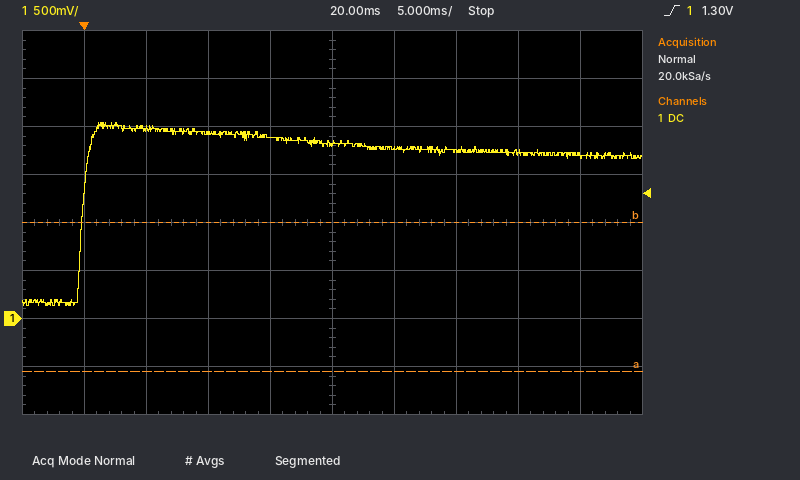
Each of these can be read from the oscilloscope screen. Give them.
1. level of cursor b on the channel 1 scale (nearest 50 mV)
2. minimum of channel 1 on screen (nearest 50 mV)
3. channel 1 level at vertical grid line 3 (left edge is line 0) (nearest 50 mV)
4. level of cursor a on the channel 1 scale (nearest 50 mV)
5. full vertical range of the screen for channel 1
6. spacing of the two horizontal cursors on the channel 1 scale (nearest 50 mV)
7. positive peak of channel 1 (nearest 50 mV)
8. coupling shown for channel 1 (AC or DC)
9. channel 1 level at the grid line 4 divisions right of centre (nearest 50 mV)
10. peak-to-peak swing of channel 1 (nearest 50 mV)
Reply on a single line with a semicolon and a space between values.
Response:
1.00 V; 150 mV; 1.95 V; -550 mV; 4 V; 1.55 V; 2.05 V; DC; 1.70 V; 1.90 V
